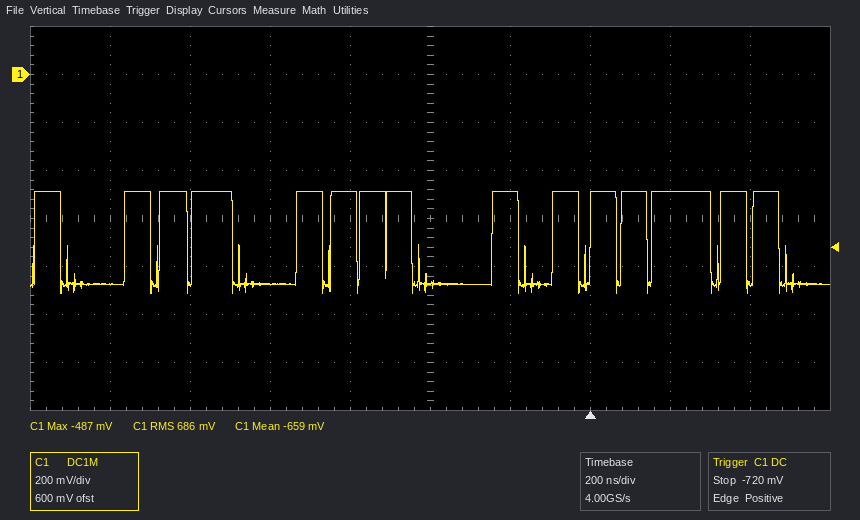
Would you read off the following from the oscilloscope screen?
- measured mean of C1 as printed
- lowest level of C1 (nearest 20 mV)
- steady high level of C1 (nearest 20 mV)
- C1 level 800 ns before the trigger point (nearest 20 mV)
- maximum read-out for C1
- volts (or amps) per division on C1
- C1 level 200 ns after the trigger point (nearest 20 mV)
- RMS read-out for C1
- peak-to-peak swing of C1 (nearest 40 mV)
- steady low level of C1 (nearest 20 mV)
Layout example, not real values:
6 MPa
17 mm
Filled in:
-659 mV
-920 mV
-480 mV
-880 mV
-487 mV
200 mV
-480 mV
686 mV
440 mV
-880 mV
